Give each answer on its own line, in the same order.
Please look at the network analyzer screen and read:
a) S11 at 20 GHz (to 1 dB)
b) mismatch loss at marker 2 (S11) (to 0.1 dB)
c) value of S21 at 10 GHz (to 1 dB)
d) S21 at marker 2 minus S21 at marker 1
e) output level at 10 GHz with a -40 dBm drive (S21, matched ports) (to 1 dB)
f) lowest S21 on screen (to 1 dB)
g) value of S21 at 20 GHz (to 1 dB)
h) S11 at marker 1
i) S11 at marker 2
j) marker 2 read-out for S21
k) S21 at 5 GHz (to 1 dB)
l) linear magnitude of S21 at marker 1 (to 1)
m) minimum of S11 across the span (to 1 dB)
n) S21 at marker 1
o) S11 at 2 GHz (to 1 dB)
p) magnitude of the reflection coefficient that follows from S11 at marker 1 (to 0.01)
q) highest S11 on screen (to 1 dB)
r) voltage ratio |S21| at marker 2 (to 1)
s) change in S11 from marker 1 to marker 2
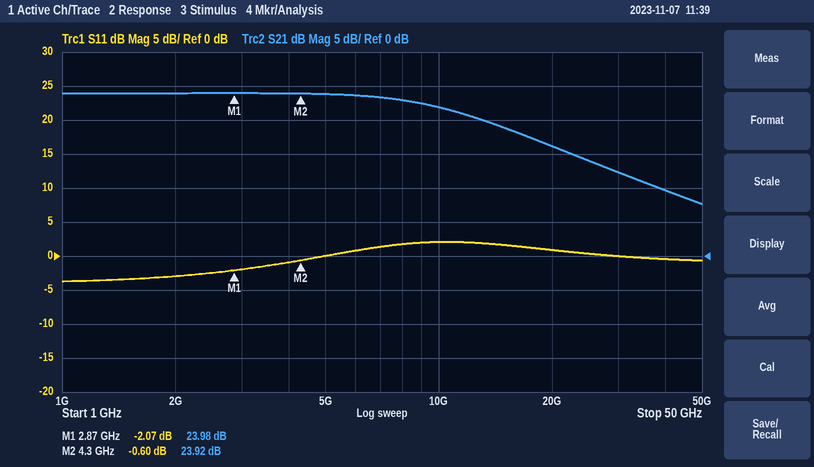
1 dB
8.9 dB
22 dB
-0.06 dB
-18 dBm
8 dB
16 dB
-2.07 dB
-0.60 dB
23.92 dB
24 dB
16
-4 dB
23.98 dB
-3 dB
0.79
2 dB
16
1.47 dB
